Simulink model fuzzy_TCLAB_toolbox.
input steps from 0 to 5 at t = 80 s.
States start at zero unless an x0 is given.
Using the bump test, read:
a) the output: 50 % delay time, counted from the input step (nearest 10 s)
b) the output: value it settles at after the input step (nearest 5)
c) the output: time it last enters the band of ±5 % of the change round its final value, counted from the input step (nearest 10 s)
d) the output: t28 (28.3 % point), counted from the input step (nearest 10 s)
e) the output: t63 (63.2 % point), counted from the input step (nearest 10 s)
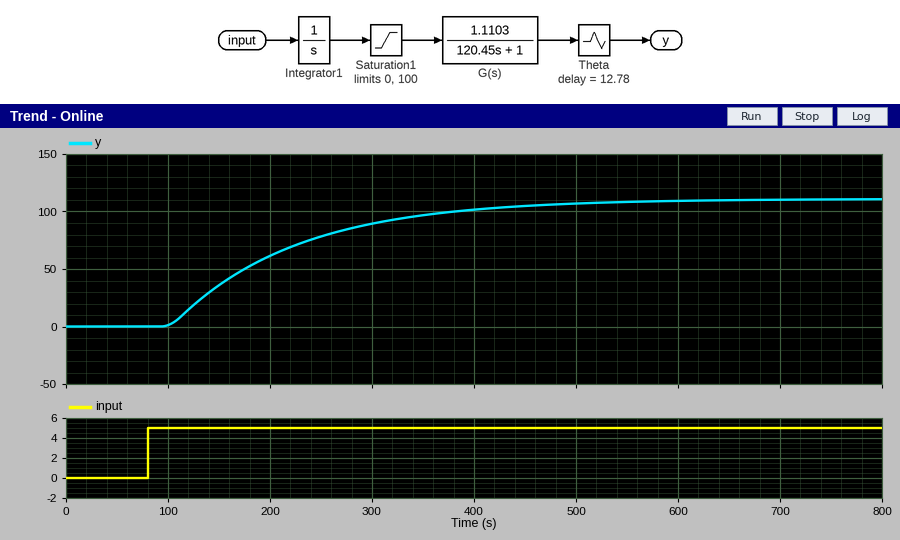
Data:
110 s
110
380 s
60 s
140 s
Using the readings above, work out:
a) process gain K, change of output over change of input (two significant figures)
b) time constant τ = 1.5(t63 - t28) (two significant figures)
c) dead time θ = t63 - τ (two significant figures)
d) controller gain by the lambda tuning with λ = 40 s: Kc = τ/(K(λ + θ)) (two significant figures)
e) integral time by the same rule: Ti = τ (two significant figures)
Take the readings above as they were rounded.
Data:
22
120 s
20 s
0.091
120 s
